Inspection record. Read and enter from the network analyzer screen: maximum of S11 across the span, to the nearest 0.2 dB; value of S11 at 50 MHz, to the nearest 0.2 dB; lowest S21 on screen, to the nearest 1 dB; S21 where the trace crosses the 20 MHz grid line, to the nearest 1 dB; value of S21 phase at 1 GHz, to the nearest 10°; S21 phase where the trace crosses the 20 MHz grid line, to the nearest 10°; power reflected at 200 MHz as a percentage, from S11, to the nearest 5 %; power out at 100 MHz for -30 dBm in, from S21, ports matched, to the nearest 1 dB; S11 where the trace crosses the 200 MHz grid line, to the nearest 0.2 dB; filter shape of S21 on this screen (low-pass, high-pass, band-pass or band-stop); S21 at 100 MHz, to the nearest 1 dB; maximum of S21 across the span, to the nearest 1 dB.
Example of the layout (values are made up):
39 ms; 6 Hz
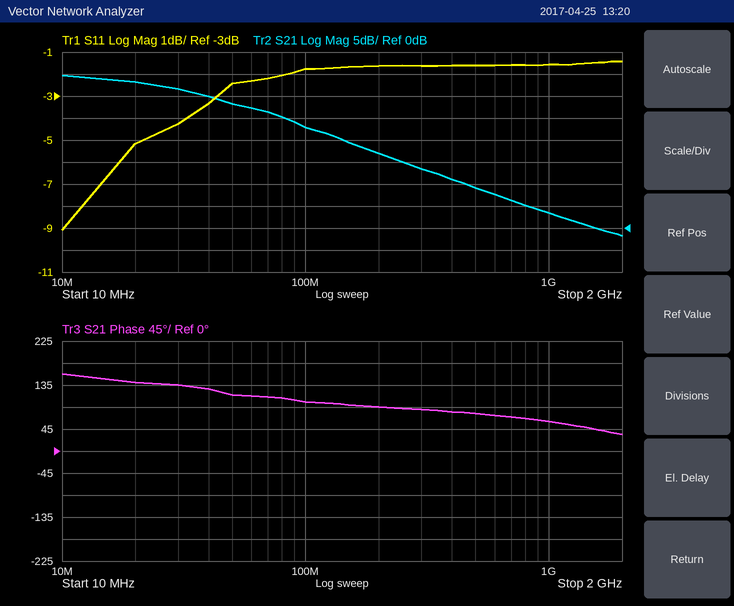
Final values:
-1.4 dB; -2.4 dB; -2 dB; 33 dB; 60°; 140°; 70 %; -7 dBm; -1.6 dB; low-pass; 23 dB; 35 dB
